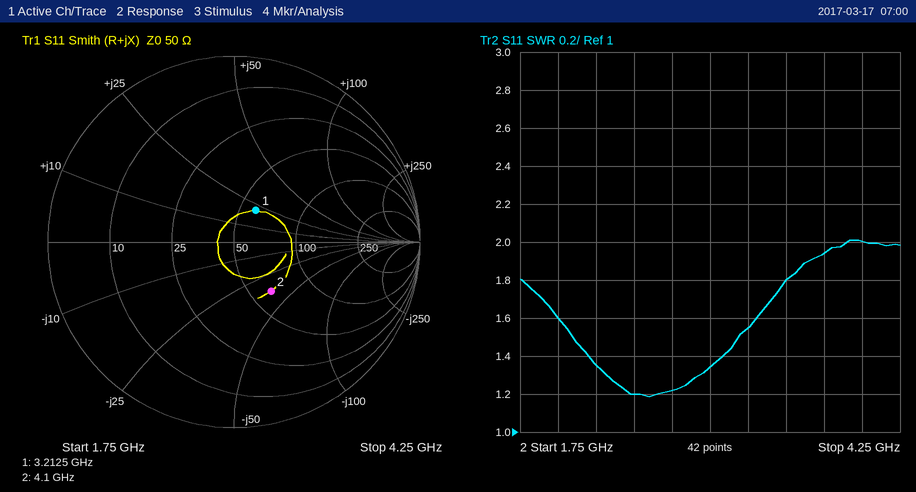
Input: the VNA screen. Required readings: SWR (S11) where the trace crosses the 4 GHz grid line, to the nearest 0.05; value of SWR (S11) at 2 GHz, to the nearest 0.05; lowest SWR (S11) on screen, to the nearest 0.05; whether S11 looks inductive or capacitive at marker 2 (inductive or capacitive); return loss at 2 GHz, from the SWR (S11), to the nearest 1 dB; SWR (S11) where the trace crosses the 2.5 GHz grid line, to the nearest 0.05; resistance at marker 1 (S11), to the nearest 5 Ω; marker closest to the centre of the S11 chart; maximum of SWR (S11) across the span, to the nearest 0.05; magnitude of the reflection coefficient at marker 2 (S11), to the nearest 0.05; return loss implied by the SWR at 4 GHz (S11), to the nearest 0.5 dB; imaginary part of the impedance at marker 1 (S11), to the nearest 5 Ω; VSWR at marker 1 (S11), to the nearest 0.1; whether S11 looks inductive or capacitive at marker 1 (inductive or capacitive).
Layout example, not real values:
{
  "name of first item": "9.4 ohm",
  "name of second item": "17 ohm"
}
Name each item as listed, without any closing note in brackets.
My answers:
{
  "SWR (S11) where the trace crosses the 4 GHz grid line, to the nearest 0.05": "2.00",
  "value of SWR (S11) at 2 GHz, to the nearest 0.05": "1.60",
  "lowest SWR (S11) on screen, to the nearest 0.05": "1.20",
  "whether S11 looks inductive or capacitive at marker 2": "capacitive",
  "return loss at 2 GHz, from the SWR (S11), to the nearest 1 dB": "13 dB",
  "SWR (S11) where the trace crosses the 2.5 GHz grid line, to the nearest 0.05": "1.20",
  "resistance at marker 1 (S11), to the nearest 5 Ω": "60 Ω",
  "marker closest to the centre of the S11 chart": "marker 1",
  "maximum of SWR (S11) across the span, to the nearest 0.05": "2.00",
  "magnitude of the reflection coefficient at marker 2 (S11), to the nearest 0.05": "0.35",
  "return loss implied by the SWR at 4 GHz (S11), to the nearest 0.5 dB": "9.5 dB",
  "imaginary part of the impedance at marker 1 (S11), to the nearest 5 Ω": "+20 Ω",
  "VSWR at marker 1 (S11), to the nearest 0.1": "1.5",
  "whether S11 looks inductive or capacitive at marker 1": "inductive"
}
